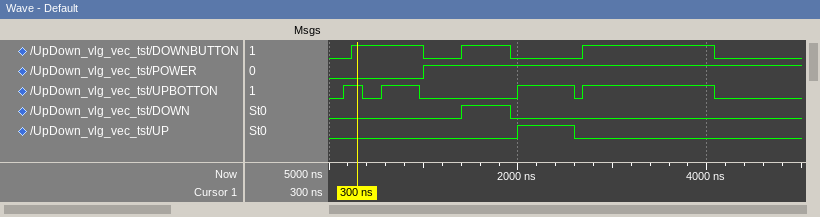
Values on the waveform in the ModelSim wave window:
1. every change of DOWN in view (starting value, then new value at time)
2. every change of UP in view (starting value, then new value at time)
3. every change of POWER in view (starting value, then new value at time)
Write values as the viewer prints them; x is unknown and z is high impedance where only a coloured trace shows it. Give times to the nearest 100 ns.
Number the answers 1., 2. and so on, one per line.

1. 0, 1 at 1400 ns, 0 at 1900 ns
2. 0, 1 at 2000 ns, 0 at 2600 ns
3. 0, 1 at 1000 ns
